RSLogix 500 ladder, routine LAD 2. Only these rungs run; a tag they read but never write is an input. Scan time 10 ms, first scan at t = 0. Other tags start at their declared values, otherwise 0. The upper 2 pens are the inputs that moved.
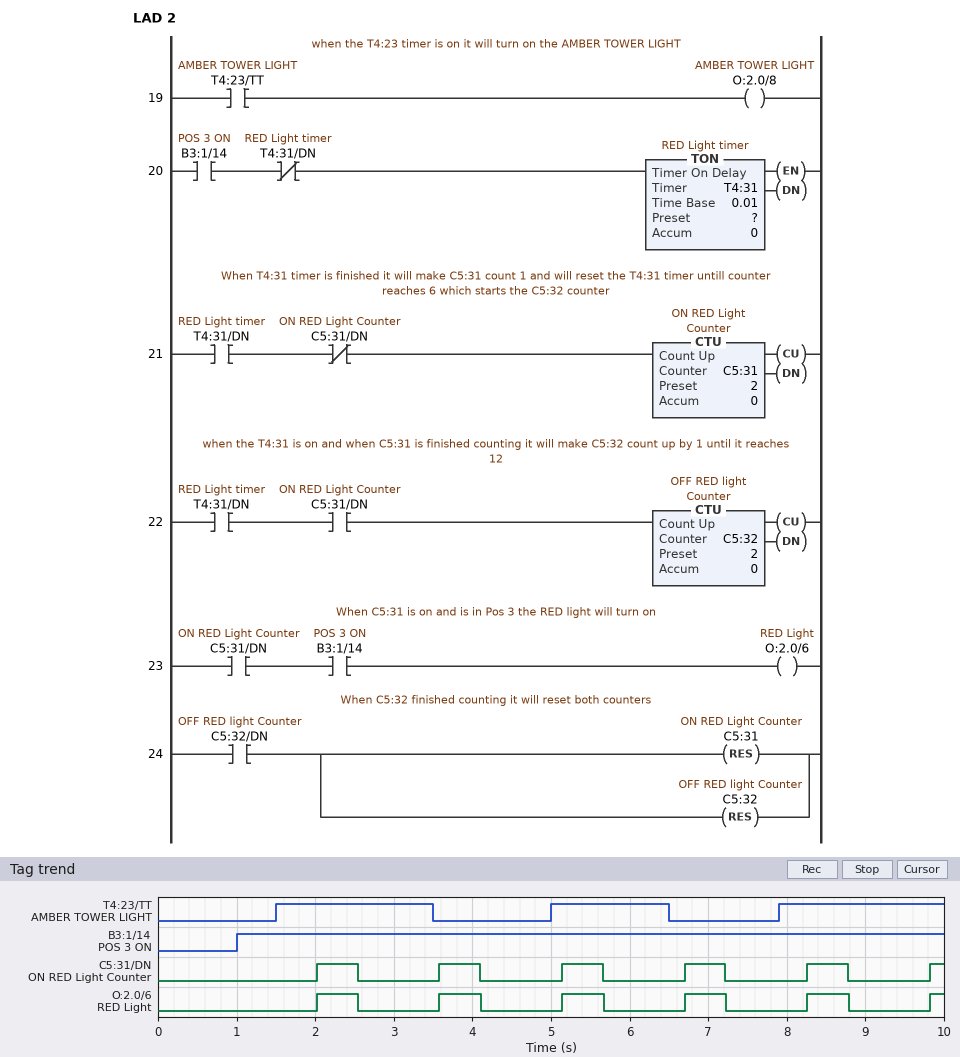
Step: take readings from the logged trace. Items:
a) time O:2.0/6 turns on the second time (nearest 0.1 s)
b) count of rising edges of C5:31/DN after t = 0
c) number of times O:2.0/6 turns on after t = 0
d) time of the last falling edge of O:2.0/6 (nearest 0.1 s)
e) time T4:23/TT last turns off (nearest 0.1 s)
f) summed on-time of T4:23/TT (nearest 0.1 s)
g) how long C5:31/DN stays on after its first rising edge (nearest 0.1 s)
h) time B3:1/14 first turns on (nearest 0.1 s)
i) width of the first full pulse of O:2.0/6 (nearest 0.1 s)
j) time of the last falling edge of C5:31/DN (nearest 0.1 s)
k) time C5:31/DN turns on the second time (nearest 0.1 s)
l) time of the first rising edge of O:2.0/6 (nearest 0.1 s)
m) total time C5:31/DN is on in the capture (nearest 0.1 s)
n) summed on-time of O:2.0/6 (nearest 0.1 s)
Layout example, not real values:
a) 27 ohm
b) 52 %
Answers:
a) 3.6 s
b) 6
c) 6
d) 8.8 s
e) 6.5 s
f) 5.6 s
g) 0.5 s
h) 1.0 s
i) 0.5 s
j) 8.8 s
k) 3.6 s
l) 2.0 s
m) 2.8 s
n) 2.8 s
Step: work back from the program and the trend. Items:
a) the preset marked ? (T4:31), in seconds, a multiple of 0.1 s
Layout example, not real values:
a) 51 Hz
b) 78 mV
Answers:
a) 0.5 s
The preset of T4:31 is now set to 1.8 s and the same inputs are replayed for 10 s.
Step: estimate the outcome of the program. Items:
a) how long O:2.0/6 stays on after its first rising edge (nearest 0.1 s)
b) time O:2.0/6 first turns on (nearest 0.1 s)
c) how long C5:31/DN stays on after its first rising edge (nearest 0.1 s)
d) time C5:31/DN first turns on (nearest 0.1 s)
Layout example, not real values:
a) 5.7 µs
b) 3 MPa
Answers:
a) 1.8 s
b) 4.6 s
c) 1.8 s
d) 4.6 s
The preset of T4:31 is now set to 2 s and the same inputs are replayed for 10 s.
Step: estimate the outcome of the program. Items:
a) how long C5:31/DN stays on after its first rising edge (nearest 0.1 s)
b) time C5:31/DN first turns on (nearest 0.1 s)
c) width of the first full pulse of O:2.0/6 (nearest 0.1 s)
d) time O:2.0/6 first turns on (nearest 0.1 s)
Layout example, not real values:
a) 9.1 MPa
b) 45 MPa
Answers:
a) 2.0 s
b) 5.0 s
c) 2.0 s
d) 5.0 s
